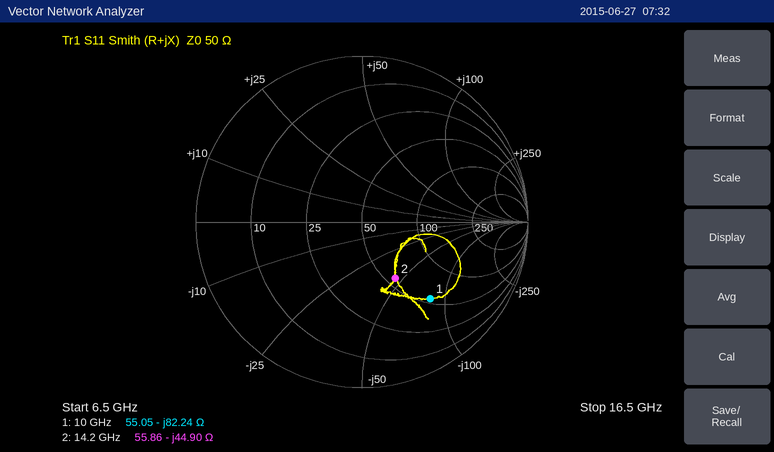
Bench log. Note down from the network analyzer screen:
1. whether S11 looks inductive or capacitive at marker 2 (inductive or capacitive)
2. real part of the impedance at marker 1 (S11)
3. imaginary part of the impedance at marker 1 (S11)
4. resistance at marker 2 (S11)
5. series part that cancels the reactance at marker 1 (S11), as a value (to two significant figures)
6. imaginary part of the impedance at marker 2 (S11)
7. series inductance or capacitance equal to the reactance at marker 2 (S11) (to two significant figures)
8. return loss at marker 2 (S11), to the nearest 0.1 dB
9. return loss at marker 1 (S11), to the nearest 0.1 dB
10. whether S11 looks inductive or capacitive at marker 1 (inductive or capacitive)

capacitive
55.05 Ω
-82.24 Ω
55.86 Ω
1.3 nH
-44.90 Ω
250 fF
8.1 dB
4.2 dB
capacitive
